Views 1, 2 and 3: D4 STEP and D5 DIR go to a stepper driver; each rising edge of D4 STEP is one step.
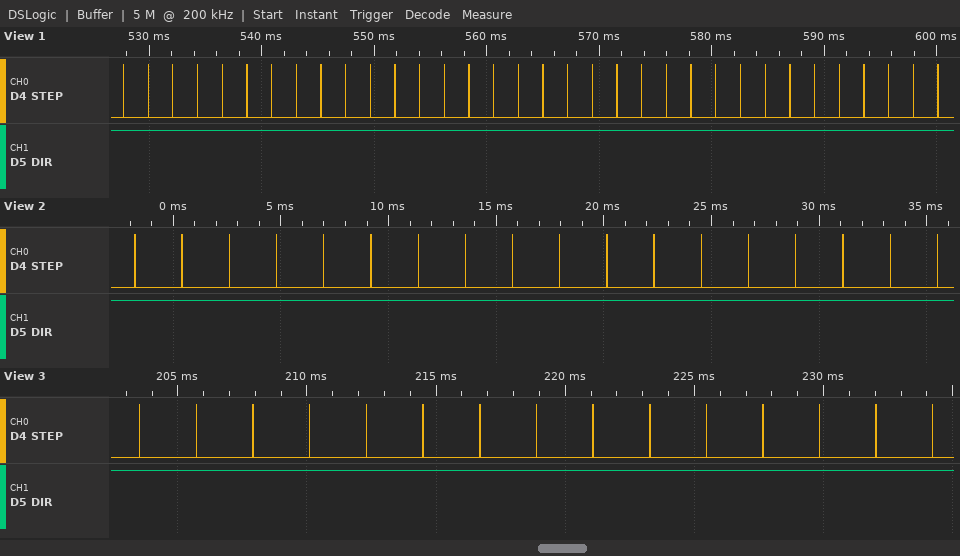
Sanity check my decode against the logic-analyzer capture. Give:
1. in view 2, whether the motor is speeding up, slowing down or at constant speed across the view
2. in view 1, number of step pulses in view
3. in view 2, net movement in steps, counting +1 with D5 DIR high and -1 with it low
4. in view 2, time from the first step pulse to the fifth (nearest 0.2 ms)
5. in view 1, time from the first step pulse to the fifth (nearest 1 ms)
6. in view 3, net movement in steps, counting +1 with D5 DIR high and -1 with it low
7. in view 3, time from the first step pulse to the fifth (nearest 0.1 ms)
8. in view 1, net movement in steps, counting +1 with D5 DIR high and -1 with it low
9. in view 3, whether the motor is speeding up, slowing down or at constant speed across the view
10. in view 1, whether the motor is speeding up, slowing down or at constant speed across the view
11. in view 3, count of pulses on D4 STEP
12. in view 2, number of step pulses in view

constant speed
34
+18
8.8 ms
9 ms
+15
8.8 ms
+34
constant speed
constant speed
15
18
